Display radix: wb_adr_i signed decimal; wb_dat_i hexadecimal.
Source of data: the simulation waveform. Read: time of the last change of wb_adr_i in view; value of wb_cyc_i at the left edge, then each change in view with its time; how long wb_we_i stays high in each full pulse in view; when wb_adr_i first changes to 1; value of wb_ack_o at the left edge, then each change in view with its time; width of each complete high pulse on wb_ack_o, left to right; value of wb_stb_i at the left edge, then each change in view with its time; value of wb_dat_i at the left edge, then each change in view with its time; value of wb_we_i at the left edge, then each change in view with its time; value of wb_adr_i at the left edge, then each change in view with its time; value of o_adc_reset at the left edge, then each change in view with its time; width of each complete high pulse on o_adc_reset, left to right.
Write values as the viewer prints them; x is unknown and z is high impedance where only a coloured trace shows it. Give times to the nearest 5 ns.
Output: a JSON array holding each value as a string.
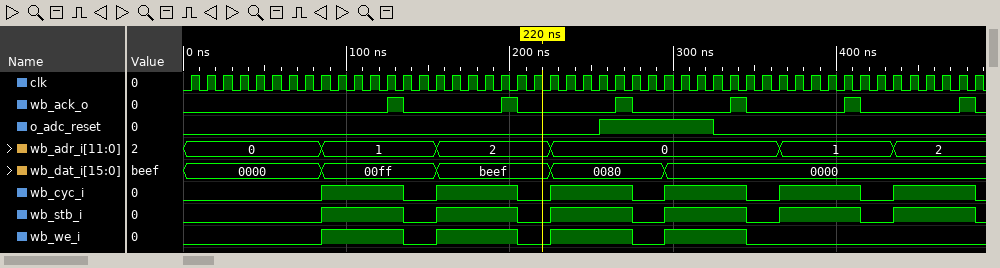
["435 ns", "0, 1 at 85 ns, 0 at 135 ns, 1 at 155 ns, 0 at 205 ns, 1 at 225 ns, 0 at 275 ns, 1 at 295 ns, 0 at 345 ns, 1 at 365 ns, 0 at 415 ns, 1 at 435 ns, 0 at 485 ns", "50 ns, 50 ns, 50 ns, 50 ns", "85 ns", "0, 1 at 125 ns, 0 at 135 ns, 1 at 195 ns, 0 at 205 ns, 1 at 265 ns, 0 at 275 ns, 1 at 335 ns, 0 at 345 ns, 1 at 405 ns, 0 at 415 ns, 1 at 475 ns, 0 at 485 ns", "10 ns, 10 ns, 10 ns, 10 ns, 10 ns, 10 ns", "0, 1 at 85 ns, 0 at 135 ns, 1 at 155 ns, 0 at 205 ns, 1 at 225 ns, 0 at 275 ns, 1 at 295 ns, 0 at 345 ns, 1 at 365 ns, 0 at 415 ns, 1 at 435 ns, 0 at 485 ns", "0000, 00ff at 85 ns, beef at 155 ns, 0080 at 225 ns, 0000 at 295 ns", "0, 1 at 85 ns, 0 at 135 ns, 1 at 155 ns, 0 at 205 ns, 1 at 225 ns, 0 at 275 ns, 1 at 295 ns, 0 at 345 ns", "0, 1 at 85 ns, 2 at 155 ns, 0 at 225 ns, 1 at 365 ns, 2 at 435 ns", "0, 1 at 255 ns, 0 at 325 ns", "70 ns"]
